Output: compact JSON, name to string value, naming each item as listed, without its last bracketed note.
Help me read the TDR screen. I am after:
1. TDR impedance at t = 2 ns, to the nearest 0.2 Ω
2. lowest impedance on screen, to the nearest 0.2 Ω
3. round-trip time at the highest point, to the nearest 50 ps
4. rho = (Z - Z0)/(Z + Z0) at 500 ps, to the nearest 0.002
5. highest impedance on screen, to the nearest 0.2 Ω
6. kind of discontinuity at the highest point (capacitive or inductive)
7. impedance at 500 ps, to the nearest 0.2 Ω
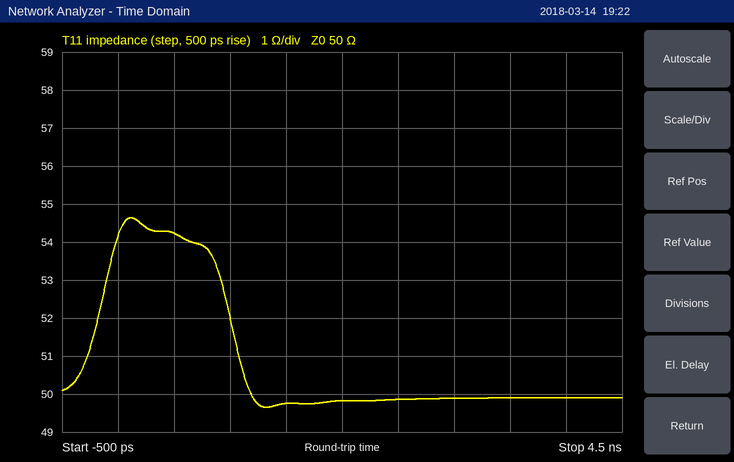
{"TDR impedance at t = 2 ns, to the nearest 0.2 Ω": "49.8 Ω", "lowest impedance on screen, to the nearest 0.2 Ω": "49.6 Ω", "round-trip time at the highest point, to the nearest 50 ps": "100 ps", "rho = (Z - Z0)/(Z + Z0) at 500 ps, to the nearest 0.002": "+0.040", "highest impedance on screen, to the nearest 0.2 Ω": "54.6 Ω", "kind of discontinuity at the highest point": "inductive", "impedance at 500 ps, to the nearest 0.2 Ω": "54.2 Ω"}
